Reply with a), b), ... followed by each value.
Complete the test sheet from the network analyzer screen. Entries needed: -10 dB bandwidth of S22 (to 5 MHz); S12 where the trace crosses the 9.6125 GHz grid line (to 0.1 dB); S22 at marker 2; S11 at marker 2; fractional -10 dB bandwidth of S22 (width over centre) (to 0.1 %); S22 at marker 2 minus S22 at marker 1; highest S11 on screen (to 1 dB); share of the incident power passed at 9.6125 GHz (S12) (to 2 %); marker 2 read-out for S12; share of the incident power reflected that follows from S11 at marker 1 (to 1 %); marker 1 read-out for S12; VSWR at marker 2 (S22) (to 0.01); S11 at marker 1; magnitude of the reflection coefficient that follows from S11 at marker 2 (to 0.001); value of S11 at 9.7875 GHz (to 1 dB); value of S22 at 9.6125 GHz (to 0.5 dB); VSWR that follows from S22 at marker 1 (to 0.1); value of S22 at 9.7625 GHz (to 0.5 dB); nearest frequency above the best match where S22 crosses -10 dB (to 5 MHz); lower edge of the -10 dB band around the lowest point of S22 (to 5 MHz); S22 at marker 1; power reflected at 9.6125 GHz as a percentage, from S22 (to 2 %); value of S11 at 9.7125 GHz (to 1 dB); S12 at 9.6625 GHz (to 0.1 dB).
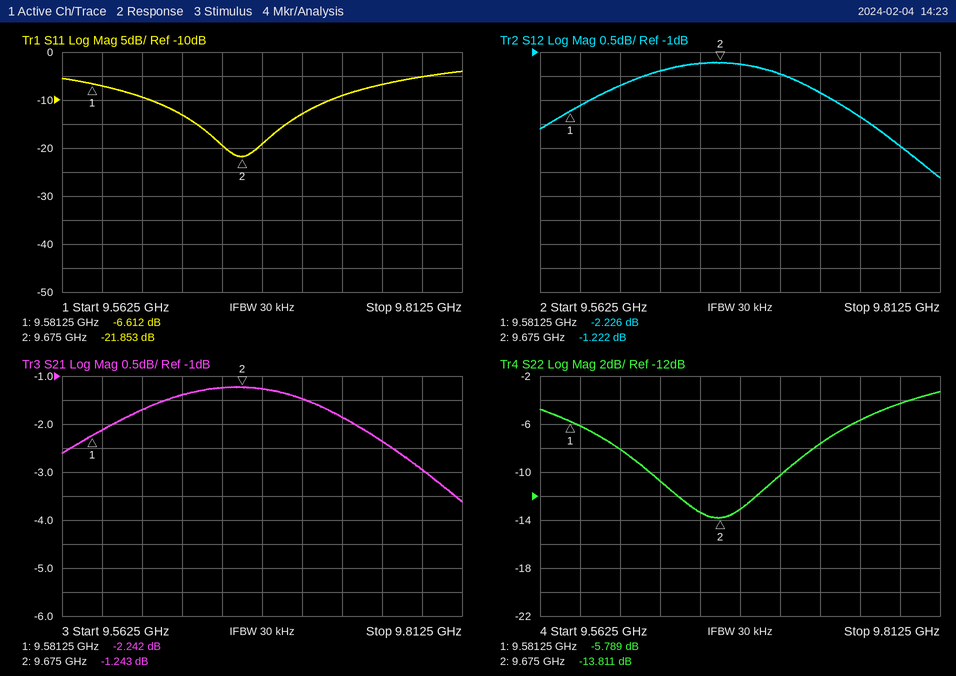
a) 85 MHz
b) -1.7 dB
c) -13.811 dB
d) -21.853 dB
e) 0.9 %
f) -8.022 dB
g) -4 dB
h) 68 %
i) -1.222 dB
j) 22 %
k) -2.226 dB
l) 1.51
m) -6.612 dB
n) 0.081
o) -5 dB
p) -8.0 dB
q) 3.1
r) -5.5 dB
s) 9.715 GHz
t) 9.630 GHz
u) -5.789 dB
v) 16 %
w) -13 dB
x) -1.2 dB
